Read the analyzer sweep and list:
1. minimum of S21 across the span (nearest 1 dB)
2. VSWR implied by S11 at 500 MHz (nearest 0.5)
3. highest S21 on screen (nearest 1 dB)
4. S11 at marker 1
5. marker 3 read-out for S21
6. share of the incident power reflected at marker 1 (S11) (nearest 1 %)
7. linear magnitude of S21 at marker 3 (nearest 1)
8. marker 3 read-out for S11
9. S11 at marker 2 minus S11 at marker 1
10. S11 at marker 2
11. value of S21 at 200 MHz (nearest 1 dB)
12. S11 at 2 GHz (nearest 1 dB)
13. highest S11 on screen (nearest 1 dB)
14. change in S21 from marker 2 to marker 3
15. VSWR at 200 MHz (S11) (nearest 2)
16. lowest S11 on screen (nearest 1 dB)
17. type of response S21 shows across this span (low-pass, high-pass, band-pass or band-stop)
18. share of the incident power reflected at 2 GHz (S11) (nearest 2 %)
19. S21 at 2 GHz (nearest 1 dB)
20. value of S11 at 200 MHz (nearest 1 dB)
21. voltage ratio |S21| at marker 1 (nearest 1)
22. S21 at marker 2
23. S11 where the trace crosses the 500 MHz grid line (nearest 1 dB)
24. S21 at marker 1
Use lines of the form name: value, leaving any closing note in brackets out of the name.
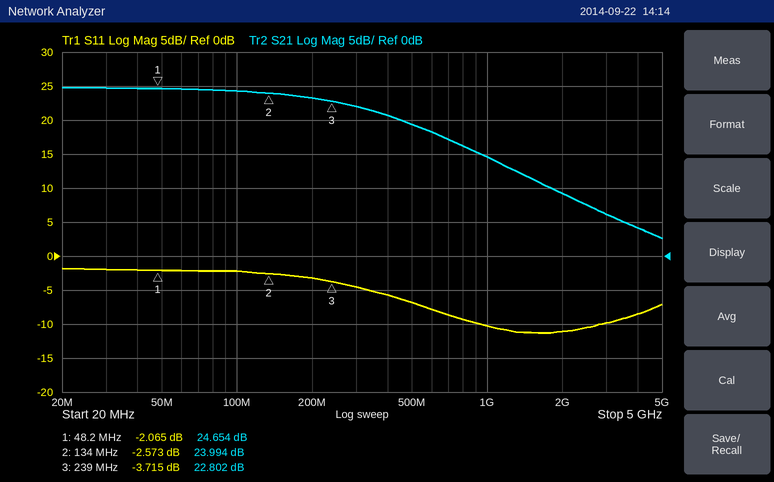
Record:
minimum of S21 across the span: 3 dB
VSWR implied by S11 at 500 MHz: 2.5
highest S21 on screen: 25 dB
S11 at marker 1: -2.065 dB
marker 3 read-out for S21: 22.802 dB
share of the incident power reflected at marker 1 (S11): 62 %
linear magnitude of S21 at marker 3: 14
marker 3 read-out for S11: -3.715 dB
S11 at marker 2 minus S11 at marker 1: -0.508 dB
S11 at marker 2: -2.573 dB
value of S21 at 200 MHz: 23 dB
S11 at 2 GHz: -11 dB
highest S11 on screen: -2 dB
change in S21 from marker 2 to marker 3: -1.192 dB
VSWR at 200 MHz (S11): 6
lowest S11 on screen: -11 dB
type of response S21 shows across this span: low-pass
share of the incident power reflected at 2 GHz (S11): 8 %
S21 at 2 GHz: 9 dB
value of S11 at 200 MHz: -3 dB
voltage ratio |S21| at marker 1: 17
S21 at marker 2: 23.994 dB
S11 where the trace crosses the 500 MHz grid line: -7 dB
S21 at marker 1: 24.654 dB
